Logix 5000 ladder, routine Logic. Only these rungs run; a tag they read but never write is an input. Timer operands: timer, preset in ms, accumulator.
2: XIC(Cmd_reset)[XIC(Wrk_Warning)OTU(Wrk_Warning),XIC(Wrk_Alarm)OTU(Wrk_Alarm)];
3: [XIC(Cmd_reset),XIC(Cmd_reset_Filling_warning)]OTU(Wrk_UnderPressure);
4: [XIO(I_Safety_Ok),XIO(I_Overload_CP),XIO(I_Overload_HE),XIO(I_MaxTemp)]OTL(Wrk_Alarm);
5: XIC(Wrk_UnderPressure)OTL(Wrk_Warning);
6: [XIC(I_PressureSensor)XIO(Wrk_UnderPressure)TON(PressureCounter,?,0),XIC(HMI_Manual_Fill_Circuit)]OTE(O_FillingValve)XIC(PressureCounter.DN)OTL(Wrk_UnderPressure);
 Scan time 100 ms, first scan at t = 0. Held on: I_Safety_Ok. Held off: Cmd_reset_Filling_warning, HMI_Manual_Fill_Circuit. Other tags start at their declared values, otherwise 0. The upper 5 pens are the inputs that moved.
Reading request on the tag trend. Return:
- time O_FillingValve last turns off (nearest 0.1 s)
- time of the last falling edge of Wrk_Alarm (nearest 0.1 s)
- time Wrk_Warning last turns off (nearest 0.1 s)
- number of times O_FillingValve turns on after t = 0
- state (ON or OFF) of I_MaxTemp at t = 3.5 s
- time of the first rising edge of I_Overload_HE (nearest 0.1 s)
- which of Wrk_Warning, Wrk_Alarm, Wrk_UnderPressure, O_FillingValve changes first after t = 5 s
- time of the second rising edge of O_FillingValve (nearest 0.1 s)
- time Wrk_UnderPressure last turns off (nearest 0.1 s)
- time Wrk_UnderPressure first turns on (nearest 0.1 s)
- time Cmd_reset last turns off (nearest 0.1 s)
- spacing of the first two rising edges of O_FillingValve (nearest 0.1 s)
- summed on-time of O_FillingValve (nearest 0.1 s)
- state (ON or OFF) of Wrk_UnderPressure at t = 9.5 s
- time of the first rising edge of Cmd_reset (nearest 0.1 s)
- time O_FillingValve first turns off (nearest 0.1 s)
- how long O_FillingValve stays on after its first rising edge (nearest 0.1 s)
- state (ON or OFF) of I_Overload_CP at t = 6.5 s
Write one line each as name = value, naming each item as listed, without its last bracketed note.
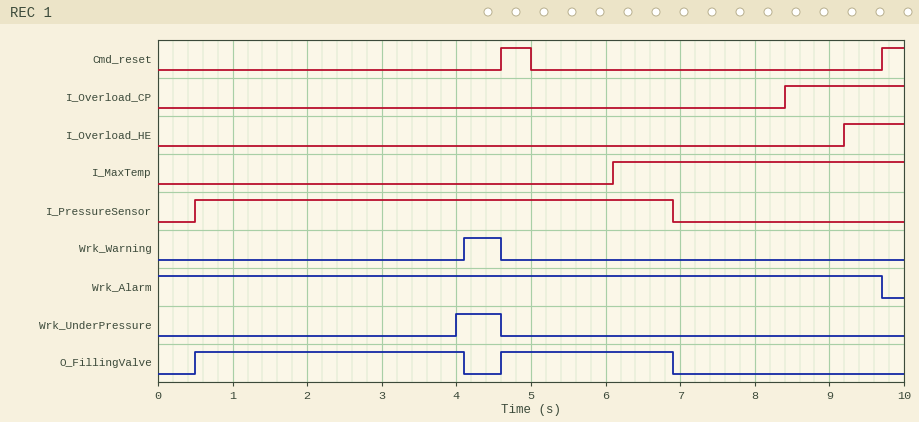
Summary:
time O_FillingValve last turns off = 6.9 s
time of the last falling edge of Wrk_Alarm = 9.7 s
time Wrk_Warning last turns off = 4.6 s
number of times O_FillingValve turns on after t = 0 = 2
state (ON or OFF) of I_MaxTemp at t = 3.5 s = OFF
time of the first rising edge of I_Overload_HE = 9.2 s
which of Wrk_Warning, Wrk_Alarm, Wrk_UnderPressure, O_FillingValve changes first after t = 5 s = O_FillingValve
time of the second rising edge of O_FillingValve = 4.6 s
time Wrk_UnderPressure last turns off = 4.6 s
time Wrk_UnderPressure first turns on = 4.0 s
time Cmd_reset last turns off = 5.0 s
spacing of the first two rising edges of O_FillingValve = 4.1 s
summed on-time of O_FillingValve = 5.9 s
state (ON or OFF) of Wrk_UnderPressure at t = 9.5 s = OFF
time of the first rising edge of Cmd_reset = 4.6 s
time O_FillingValve first turns off = 4.1 s
how long O_FillingValve stays on after its first rising edge = 3.6 s
state (ON or OFF) of I_Overload_CP at t = 6.5 s = OFF
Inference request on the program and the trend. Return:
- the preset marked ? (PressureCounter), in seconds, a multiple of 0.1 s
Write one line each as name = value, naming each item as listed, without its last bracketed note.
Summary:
the preset marked ? (PressureCounter), in seconds, a multiple of 0.1 s = 3.5 s
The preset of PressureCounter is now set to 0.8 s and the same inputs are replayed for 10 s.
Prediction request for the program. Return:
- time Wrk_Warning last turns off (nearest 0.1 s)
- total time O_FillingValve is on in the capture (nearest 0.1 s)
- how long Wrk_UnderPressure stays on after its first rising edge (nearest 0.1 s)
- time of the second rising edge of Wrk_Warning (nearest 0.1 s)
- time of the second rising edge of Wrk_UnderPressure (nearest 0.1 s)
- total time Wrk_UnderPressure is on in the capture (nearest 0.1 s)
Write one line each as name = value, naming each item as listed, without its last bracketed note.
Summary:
time Wrk_Warning last turns off = 9.7 s
total time O_FillingValve is on in the capture = 1.8 s
how long Wrk_UnderPressure stays on after its first rising edge = 3.3 s
time of the second rising edge of Wrk_Warning = 5.5 s
time of the second rising edge of Wrk_UnderPressure = 5.4 s
total time Wrk_UnderPressure is on in the capture = 7.6 s
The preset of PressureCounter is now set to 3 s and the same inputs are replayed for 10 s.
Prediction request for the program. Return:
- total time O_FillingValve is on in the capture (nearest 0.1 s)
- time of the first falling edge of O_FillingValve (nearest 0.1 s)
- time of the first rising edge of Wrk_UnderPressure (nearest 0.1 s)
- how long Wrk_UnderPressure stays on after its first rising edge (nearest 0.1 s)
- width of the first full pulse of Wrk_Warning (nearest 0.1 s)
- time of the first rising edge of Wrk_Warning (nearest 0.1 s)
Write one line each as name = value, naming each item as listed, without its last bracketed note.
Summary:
total time O_FillingValve is on in the capture = 5.4 s
time of the first falling edge of O_FillingValve = 3.6 s
time of the first rising edge of Wrk_UnderPressure = 3.5 s
how long Wrk_UnderPressure stays on after its first rising edge = 1.1 s
width of the first full pulse of Wrk_Warning = 1.0 s
time of the first rising edge of Wrk_Warning = 3.6 s
